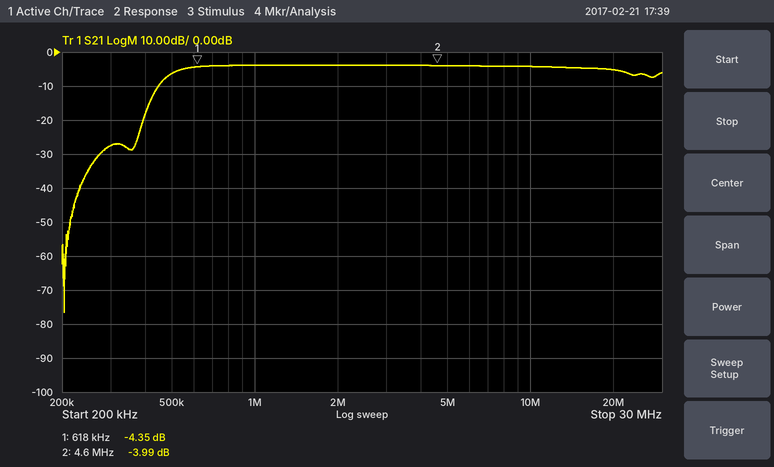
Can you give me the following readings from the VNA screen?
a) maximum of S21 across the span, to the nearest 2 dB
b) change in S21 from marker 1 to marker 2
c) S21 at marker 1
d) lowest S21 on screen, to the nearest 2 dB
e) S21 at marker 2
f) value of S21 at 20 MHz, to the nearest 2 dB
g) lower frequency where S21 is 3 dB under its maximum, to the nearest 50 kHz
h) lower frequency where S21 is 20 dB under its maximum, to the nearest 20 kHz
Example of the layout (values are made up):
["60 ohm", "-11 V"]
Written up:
["-4 dB", "0.36 dB", "-4.35 dB", "-76 dB", "-3.99 dB", "-6 dB", "500 kHz", "380 kHz"]
